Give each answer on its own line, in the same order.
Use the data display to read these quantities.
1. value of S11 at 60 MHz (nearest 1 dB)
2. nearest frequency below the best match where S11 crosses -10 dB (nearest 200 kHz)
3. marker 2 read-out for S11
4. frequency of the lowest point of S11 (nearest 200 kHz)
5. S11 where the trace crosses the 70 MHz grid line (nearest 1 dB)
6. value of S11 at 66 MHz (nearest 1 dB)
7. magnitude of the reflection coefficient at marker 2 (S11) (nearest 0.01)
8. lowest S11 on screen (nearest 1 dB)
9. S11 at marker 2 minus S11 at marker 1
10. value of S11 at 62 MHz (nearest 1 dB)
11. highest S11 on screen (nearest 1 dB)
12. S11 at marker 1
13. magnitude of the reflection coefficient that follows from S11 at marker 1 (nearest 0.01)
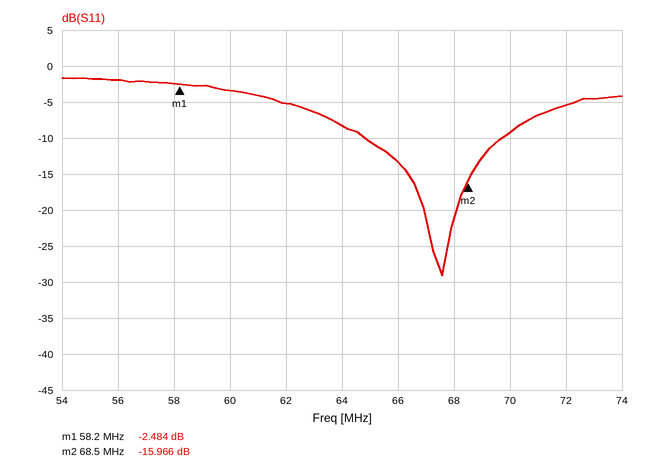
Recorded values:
-3 dB
64.8 MHz
-15.966 dB
67.6 MHz
-9 dB
-13 dB
0.16
-29 dB
-13.482 dB
-5 dB
-2 dB
-2.484 dB
0.75
